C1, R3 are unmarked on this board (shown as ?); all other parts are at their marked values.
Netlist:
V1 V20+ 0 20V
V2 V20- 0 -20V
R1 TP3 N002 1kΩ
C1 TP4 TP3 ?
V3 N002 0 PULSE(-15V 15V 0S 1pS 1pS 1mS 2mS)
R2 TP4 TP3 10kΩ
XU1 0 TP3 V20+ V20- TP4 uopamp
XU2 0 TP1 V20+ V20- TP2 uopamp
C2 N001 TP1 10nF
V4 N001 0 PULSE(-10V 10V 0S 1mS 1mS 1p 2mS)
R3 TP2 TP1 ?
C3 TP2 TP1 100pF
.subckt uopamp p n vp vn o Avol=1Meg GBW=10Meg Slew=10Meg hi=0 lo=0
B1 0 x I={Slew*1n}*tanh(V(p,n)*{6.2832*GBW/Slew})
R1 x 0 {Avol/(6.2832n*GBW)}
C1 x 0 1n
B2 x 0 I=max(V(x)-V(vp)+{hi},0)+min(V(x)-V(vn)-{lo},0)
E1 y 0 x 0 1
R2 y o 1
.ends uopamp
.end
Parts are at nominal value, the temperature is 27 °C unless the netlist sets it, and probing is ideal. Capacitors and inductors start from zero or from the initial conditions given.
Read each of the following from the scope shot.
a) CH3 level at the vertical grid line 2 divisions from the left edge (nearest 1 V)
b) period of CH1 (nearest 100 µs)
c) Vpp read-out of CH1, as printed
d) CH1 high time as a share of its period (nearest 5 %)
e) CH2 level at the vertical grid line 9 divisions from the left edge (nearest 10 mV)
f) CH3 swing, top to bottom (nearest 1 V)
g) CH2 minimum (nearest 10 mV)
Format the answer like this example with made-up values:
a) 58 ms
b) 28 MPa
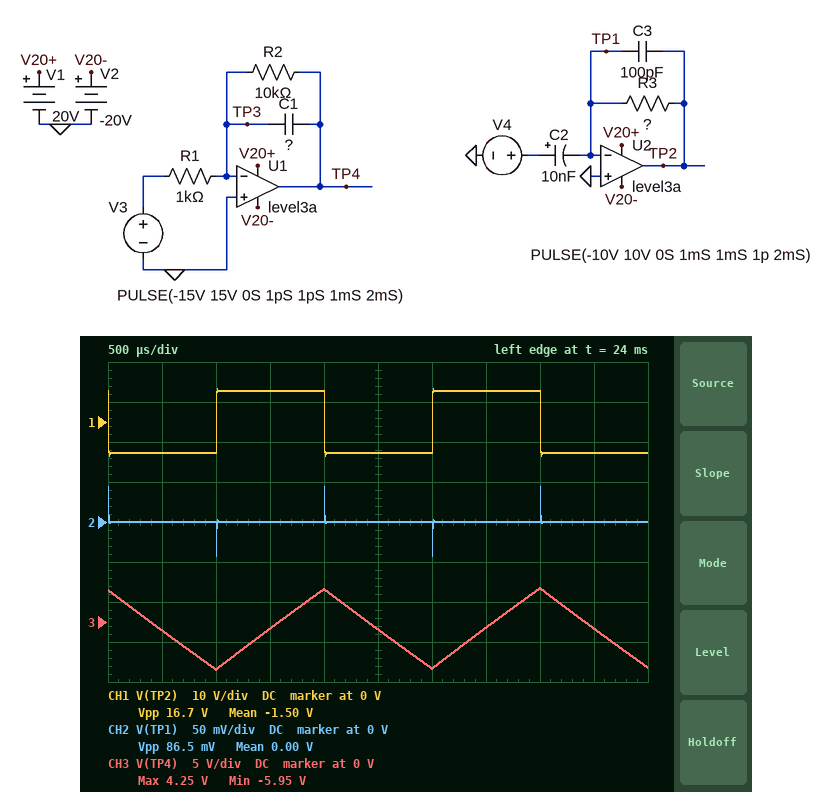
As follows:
a) -6 V
b) 2.0 ms
c) 16.7 V
d) 50 %
e) 0 V
f) 10 V
g) -40 mV
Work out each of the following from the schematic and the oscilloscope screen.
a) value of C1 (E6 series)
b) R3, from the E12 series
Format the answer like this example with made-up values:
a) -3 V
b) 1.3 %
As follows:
a) 1.5 µF
b) 39 kΩ
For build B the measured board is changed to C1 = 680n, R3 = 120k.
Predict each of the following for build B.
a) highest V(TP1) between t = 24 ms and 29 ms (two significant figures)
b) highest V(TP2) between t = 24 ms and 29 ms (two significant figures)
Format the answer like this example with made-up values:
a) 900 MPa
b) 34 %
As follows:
a) 2.1 V
b) 20 V
